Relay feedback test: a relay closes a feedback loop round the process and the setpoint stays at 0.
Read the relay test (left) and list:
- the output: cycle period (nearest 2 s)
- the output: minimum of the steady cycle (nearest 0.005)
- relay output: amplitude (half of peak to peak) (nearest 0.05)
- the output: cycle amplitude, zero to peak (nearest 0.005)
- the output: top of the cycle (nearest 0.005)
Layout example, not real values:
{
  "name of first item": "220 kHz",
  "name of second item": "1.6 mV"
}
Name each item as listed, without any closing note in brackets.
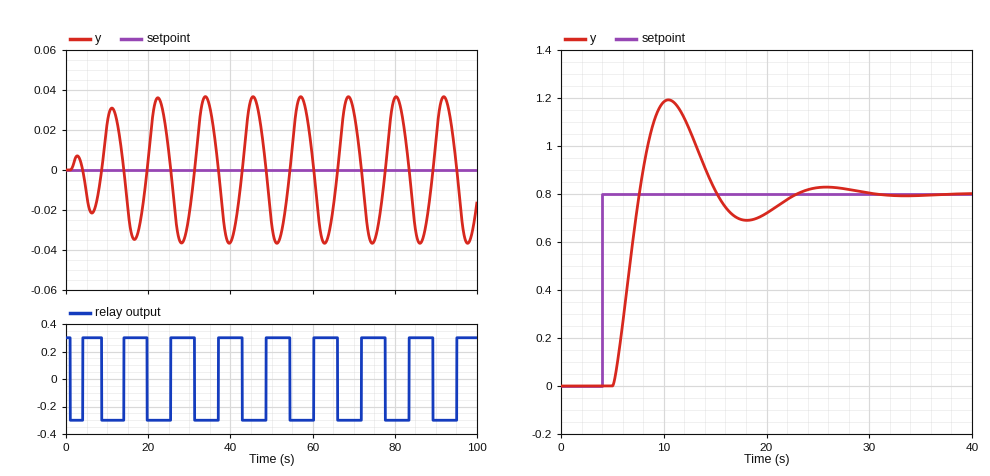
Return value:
{
  "the output: cycle period": "12 s",
  "the output: minimum of the steady cycle": "-0.035",
  "relay output: amplitude (half of peak to peak)": "0.30",
  "the output: cycle amplitude, zero to peak": "0.035",
  "the output: top of the cycle": "0.035"
}
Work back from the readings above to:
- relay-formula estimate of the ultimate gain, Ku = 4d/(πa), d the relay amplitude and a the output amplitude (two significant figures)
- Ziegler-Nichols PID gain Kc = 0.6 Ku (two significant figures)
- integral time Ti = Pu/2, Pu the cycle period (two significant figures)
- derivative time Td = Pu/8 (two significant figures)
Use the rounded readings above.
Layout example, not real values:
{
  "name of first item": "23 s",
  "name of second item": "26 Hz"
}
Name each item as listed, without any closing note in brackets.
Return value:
{
  "relay-formula estimate of the ultimate gain, Ku = 4d/(πa), d the relay amplitude and a the output amplitude": "11",
  "Ziegler-Nichols PID gain Kc = 0.6 Ku": "6.6",
  "integral time Ti = Pu/2, Pu the cycle period": "6.0 s",
  "derivative time Td = Pu/8": "1.5 s"
}
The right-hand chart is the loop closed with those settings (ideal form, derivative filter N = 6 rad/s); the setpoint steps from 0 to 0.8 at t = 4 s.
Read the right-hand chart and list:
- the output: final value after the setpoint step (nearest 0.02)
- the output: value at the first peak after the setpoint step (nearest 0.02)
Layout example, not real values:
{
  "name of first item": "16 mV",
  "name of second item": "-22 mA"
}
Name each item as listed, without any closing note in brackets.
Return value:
{
  "the output: final value after the setpoint step": "0.80",
  "the output: value at the first peak after the setpoint step": "1.20"
}
